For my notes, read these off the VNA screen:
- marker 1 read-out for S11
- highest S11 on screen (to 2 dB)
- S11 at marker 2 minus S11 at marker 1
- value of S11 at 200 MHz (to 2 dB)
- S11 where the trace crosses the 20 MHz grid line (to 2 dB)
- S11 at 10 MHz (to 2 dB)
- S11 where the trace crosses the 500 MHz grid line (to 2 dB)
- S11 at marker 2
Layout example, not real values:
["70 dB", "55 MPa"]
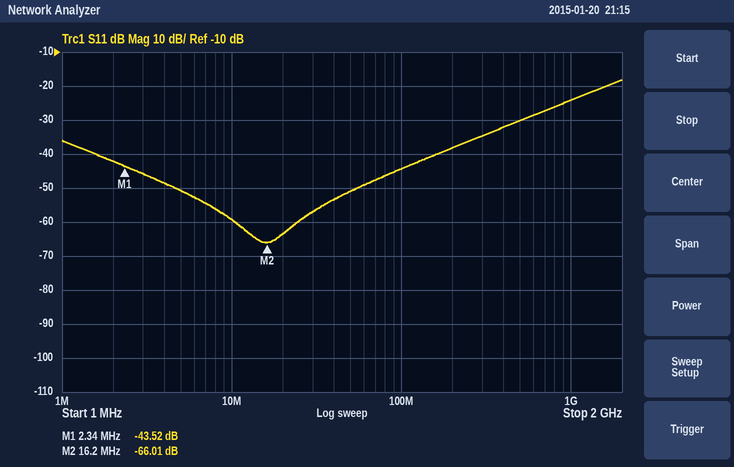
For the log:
["-43.52 dB", "-18 dB", "-22.49 dB", "-38 dB", "-64 dB", "-60 dB", "-30 dB", "-66.01 dB"]
